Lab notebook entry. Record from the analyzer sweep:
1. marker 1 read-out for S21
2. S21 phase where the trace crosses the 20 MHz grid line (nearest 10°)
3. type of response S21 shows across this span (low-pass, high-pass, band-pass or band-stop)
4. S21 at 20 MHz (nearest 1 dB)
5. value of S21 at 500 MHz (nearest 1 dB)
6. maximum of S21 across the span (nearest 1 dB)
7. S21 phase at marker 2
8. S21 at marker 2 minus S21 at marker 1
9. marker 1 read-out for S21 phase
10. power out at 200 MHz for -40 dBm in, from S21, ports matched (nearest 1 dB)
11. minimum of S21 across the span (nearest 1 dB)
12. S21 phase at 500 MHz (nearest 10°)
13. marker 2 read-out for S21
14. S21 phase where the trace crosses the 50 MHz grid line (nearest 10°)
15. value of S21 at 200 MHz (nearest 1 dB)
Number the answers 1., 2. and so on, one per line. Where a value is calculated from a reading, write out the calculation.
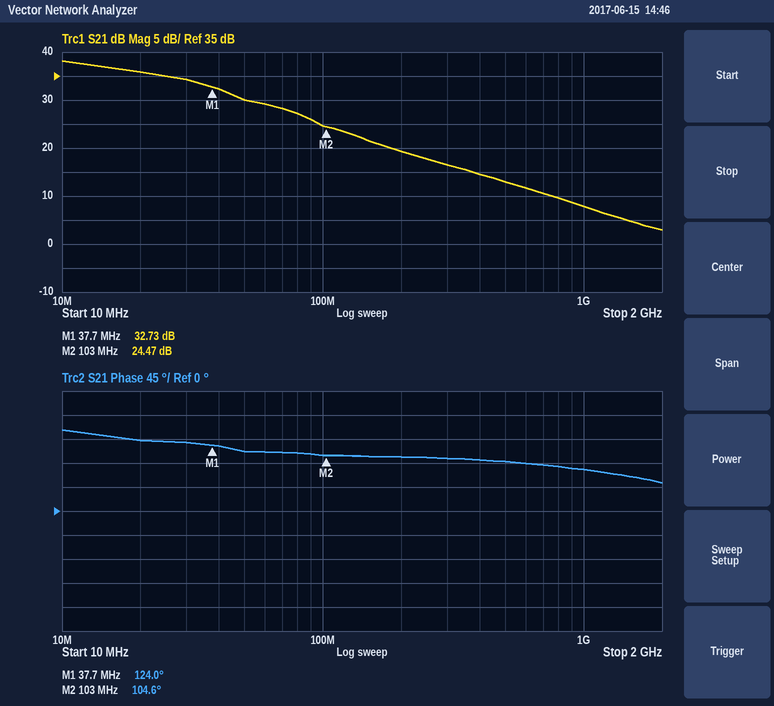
1. 32.73 dB
2. 130°
3. low-pass
4. 36 dB
5. 13 dB
6. 38 dB
7. 104.6°
8. 24.47 − (32.73) = -8.26 dB
9. 124.0°
10. -40 dBm + (19 dB) = -21 dBm
11. 3 dB
12. 90°
13. 24.47 dB
14. 110°
15. 19 dB
